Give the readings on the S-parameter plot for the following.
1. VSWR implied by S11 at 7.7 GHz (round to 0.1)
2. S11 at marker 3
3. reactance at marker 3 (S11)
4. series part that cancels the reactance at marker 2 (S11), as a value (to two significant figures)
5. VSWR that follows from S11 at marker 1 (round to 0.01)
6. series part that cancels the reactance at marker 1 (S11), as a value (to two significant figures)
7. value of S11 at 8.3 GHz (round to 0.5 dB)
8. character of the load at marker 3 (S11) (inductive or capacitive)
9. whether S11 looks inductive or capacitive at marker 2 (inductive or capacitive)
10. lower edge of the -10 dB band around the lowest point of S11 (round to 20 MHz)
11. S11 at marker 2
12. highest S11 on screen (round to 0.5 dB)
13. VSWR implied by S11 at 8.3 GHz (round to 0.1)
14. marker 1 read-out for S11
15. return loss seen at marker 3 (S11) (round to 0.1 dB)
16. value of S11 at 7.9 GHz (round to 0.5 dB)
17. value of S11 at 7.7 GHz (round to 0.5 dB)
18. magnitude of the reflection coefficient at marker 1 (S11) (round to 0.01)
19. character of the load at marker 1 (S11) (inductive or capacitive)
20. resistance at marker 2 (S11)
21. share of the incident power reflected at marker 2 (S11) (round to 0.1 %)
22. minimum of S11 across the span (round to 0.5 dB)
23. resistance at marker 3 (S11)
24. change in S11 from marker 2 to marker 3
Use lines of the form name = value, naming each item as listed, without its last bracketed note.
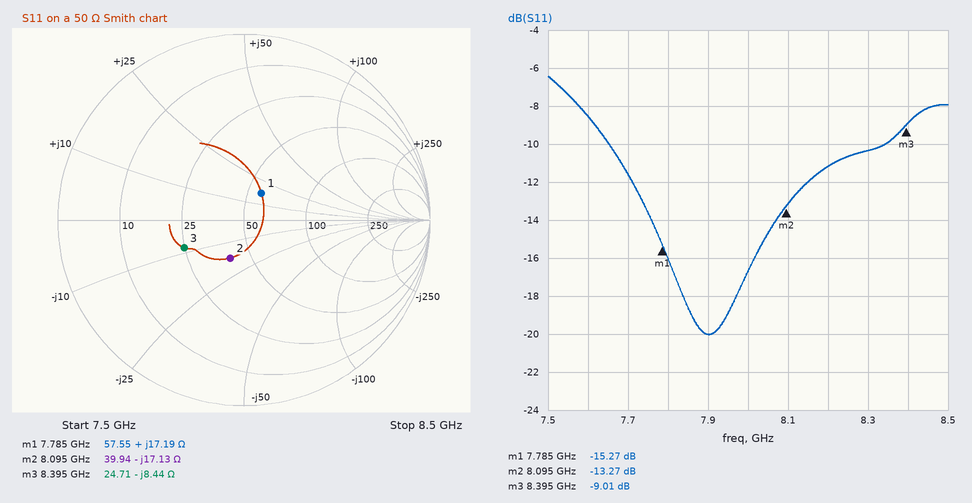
VSWR implied by S11 at 7.7 GHz = 1.7
S11 at marker 3 = -9.01 dB
reactance at marker 3 = -8.44 Ω
series part that cancels the reactance at marker 2 (S11), as a value = 340 pH
VSWR that follows from S11 at marker 1 = 1.42
series part that cancels the reactance at marker 1 (S11), as a value = 1.2 pF
value of S11 at 8.3 GHz = -10.5 dB
character of the load at marker 3 (S11) = capacitive
whether S11 looks inductive or capacitive at marker 2 = capacitive
lower edge of the -10 dB band around the lowest point of S11 = 7.66 GHz
S11 at marker 2 = -13.27 dB
highest S11 on screen = -6.5 dB
VSWR implied by S11 at 8.3 GHz = 1.9
marker 1 read-out for S11 = -15.27 dB
return loss seen at marker 3 (S11) = 9.0 dB
value of S11 at 7.9 GHz = -20.0 dB
value of S11 at 7.7 GHz = -11.5 dB
magnitude of the reflection coefficient at marker 1 (S11) = 0.17
character of the load at marker 1 (S11) = inductive
resistance at marker 2 = 39.94 Ω
share of the incident power reflected at marker 2 (S11) = 4.7 %
minimum of S11 across the span = -20.0 dB
resistance at marker 3 = 24.71 Ω
change in S11 from marker 2 to marker 3 = 4.26 dB
